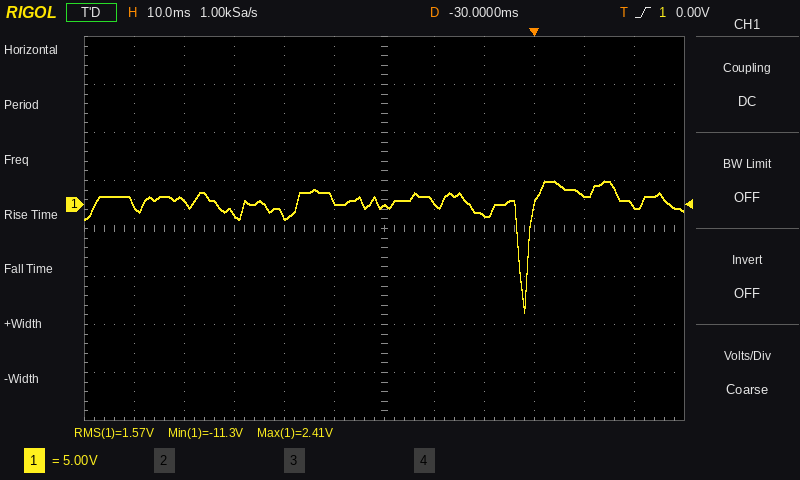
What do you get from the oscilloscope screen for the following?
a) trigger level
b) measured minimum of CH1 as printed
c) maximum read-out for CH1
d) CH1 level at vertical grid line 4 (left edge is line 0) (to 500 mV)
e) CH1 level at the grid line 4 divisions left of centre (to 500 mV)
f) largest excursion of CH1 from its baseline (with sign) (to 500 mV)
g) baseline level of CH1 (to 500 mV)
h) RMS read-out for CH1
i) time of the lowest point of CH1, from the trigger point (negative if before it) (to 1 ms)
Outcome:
0.00 V
-11.3 V
2.41 V
-1.0 V
500 mV
-11.5 V
500 mV
1.57 V
-2 ms
